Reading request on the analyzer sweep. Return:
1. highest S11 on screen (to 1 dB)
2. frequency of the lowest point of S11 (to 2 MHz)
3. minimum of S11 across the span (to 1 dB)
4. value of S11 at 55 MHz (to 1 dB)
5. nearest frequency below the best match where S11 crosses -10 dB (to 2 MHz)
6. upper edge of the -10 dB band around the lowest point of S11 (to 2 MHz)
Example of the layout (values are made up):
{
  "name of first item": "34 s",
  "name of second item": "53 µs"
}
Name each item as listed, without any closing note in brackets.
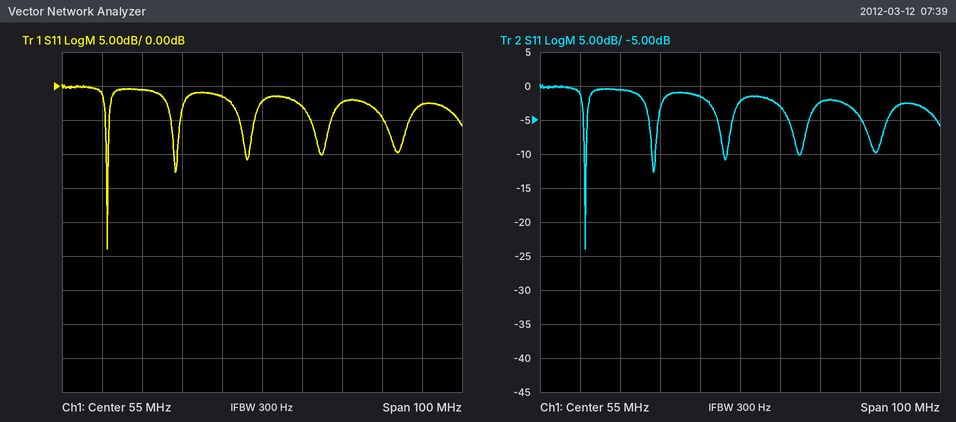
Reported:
{
  "highest S11 on screen": "0 dB",
  "frequency of the lowest point of S11": "16 MHz",
  "minimum of S11 across the span": "-24 dB",
  "value of S11 at 55 MHz": "-2 dB",
  "nearest frequency below the best match where S11 crosses -10 dB": "16 MHz",
  "upper edge of the -10 dB band around the lowest point of S11": "16 MHz"
}
